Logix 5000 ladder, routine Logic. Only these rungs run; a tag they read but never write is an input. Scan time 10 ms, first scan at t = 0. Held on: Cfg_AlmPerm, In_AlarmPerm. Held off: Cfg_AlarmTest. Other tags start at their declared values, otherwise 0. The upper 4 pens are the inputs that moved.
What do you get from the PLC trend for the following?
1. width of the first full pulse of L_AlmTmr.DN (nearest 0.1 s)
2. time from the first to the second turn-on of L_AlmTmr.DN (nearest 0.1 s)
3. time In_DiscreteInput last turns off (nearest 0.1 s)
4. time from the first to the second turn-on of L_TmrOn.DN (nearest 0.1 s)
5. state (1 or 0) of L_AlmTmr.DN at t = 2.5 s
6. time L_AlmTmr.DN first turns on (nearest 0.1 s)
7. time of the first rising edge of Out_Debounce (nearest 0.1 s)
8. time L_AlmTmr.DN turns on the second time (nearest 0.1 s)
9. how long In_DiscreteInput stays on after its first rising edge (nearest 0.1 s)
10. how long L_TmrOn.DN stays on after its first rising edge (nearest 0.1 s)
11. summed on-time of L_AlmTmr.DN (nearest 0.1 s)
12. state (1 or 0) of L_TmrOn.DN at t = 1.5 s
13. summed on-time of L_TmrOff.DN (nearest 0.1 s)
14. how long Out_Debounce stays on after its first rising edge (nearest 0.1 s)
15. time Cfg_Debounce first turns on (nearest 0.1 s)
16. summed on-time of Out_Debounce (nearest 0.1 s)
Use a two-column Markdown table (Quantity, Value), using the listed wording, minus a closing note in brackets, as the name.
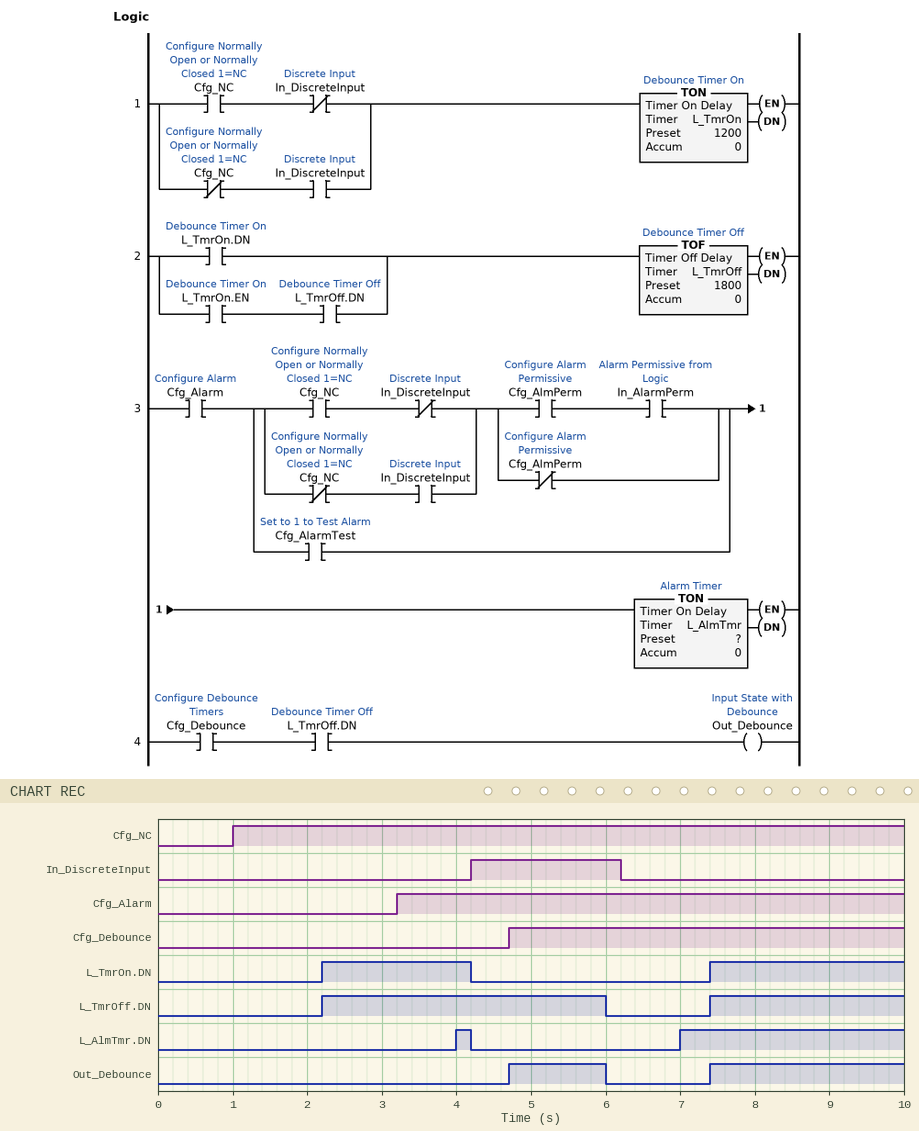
| Quantity | Value |
|---|---|
| width of the first full pulse of L_AlmTmr.DN | 0.2 s |
| time from the first to the second turn-on of L_AlmTmr.DN | 3.0 s |
| time In_DiscreteInput last turns off | 6.2 s |
| time from the first to the second turn-on of L_TmrOn.DN | 5.2 s |
| state (1 or 0) of L_AlmTmr.DN at t = 2.5 s | 0 |
| time L_AlmTmr.DN first turns on | 4.0 s |
| time of the first rising edge of Out_Debounce | 4.7 s |
| time L_AlmTmr.DN turns on the second time | 7.0 s |
| how long In_DiscreteInput stays on after its first rising edge | 2.0 s |
| how long L_TmrOn.DN stays on after its first rising edge | 2.0 s |
| summed on-time of L_AlmTmr.DN | 3.2 s |
| state (1 or 0) of L_TmrOn.DN at t = 1.5 s | 0 |
| summed on-time of L_TmrOff.DN | 6.4 s |
| how long Out_Debounce stays on after its first rising edge | 1.3 s |
| time Cfg_Debounce first turns on | 4.7 s |
| summed on-time of Out_Debounce | 3.9 s |
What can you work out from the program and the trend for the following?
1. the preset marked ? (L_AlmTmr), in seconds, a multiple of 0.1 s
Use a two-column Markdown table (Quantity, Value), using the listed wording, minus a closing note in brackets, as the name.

| Quantity | Value |
|---|---|
| the preset marked ? (L_AlmTmr), in seconds, a multiple of 0.1 s | 0.8 s |
